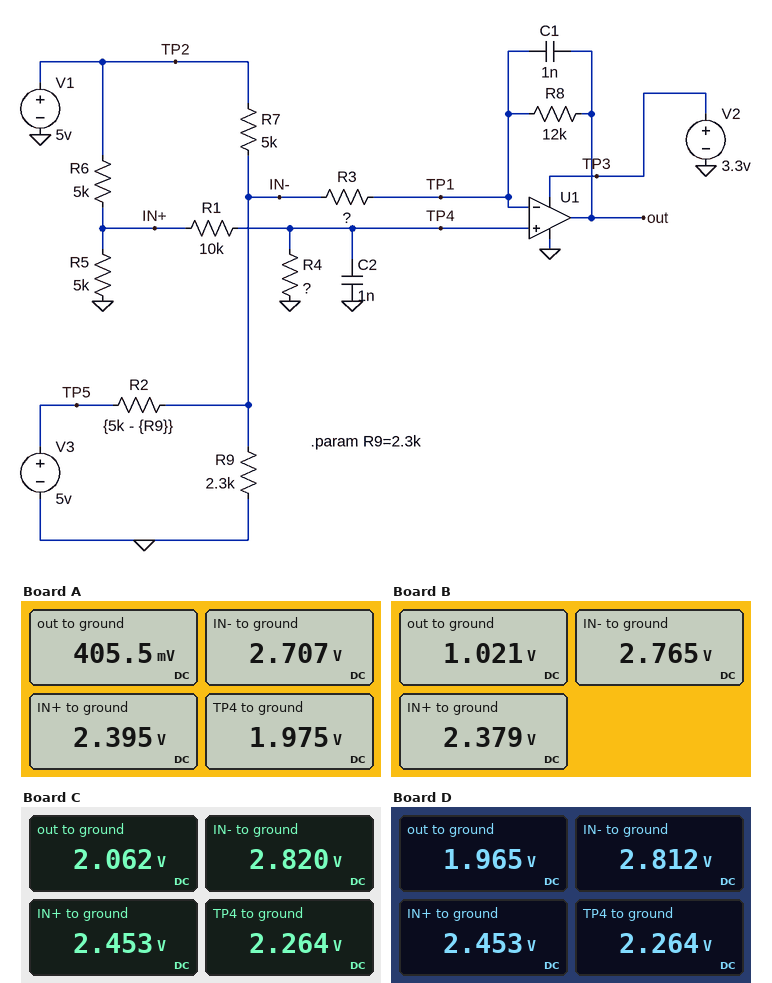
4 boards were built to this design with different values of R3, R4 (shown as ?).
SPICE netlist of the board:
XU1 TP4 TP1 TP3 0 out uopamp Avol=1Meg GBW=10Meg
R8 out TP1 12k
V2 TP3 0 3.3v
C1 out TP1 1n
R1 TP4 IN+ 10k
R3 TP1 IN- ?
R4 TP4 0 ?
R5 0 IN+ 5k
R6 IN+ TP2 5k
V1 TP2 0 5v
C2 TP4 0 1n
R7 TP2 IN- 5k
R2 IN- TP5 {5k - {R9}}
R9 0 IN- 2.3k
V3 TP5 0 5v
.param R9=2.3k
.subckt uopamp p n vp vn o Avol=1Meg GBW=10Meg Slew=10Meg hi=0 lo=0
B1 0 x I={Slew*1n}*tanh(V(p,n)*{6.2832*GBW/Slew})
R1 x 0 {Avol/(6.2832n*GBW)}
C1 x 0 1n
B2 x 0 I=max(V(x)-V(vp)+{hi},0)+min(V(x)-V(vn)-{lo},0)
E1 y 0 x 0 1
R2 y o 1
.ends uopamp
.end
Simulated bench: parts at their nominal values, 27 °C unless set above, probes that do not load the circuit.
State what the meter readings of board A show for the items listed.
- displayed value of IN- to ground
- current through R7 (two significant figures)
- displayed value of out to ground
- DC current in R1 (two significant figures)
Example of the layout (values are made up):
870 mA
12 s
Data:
2.707 V
460 µA
405.5 mV
42 µA
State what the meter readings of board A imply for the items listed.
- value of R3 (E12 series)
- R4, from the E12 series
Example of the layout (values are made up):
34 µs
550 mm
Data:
5.6 kΩ
47 kΩ
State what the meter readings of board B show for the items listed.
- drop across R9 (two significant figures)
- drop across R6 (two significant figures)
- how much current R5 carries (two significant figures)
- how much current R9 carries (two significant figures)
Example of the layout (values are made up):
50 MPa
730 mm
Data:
2.8 V
2.6 V
480 µA
1.2 mA
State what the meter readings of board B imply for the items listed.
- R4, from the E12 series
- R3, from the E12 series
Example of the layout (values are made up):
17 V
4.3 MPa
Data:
39 kΩ
12 kΩ
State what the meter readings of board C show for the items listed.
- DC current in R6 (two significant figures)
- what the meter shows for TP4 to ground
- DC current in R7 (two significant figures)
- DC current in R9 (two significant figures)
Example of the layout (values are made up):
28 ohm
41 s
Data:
510 µA
2.264 V
440 µA
1.2 mA
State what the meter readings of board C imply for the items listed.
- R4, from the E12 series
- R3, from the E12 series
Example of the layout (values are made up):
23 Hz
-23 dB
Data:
120 kΩ
33 kΩ
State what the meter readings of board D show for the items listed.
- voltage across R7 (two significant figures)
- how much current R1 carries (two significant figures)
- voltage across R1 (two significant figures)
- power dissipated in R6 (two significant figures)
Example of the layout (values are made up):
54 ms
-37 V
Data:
2.2 V
19 µA
190 mV
1.3 mW
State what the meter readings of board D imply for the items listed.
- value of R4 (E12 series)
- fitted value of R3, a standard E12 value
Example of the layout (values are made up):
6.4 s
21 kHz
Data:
120 kΩ
22 kΩ
